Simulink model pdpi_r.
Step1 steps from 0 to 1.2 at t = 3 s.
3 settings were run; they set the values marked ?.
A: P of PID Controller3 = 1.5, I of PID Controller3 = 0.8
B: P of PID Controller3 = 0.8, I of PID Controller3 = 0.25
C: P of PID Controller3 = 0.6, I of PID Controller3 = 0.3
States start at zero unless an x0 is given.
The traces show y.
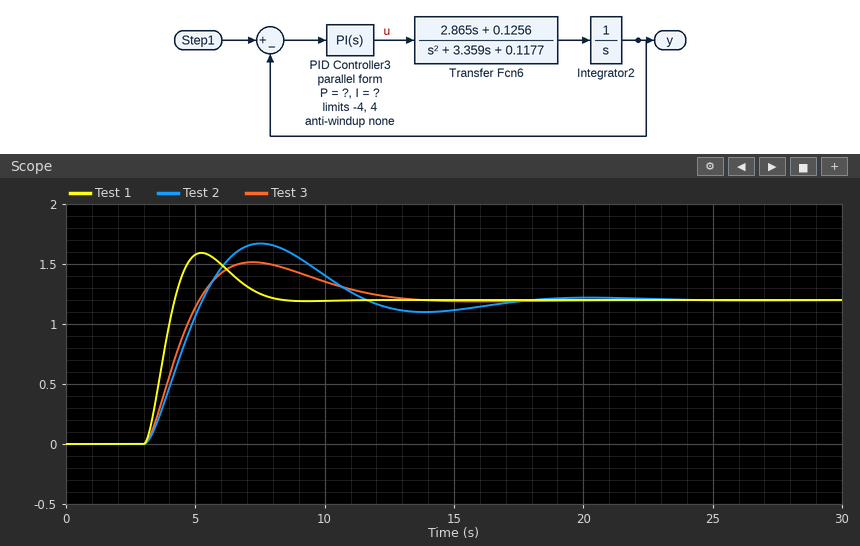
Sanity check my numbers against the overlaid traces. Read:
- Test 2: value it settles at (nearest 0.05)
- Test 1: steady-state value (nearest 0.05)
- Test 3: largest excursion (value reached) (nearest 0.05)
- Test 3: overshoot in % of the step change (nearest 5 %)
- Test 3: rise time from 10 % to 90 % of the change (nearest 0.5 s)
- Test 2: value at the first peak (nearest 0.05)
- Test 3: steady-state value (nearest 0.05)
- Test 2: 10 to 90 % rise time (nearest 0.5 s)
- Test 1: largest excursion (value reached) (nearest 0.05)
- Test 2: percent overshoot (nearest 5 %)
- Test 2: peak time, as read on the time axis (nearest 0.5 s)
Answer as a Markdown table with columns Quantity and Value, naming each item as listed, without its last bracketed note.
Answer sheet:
| Quantity | Value |
|---|---|
| Test 2: value it settles at | 1.20 |
| Test 1: steady-state value | 1.20 |
| Test 3: largest excursion (value reached) | 1.50 |
| Test 3: overshoot in % of the step change | 25 % |
| Test 3: rise time from 10 % to 90 % of the change | 1.5 s |
| Test 2: value at the first peak | 1.65 |
| Test 3: steady-state value | 1.20 |
| Test 2: 10 to 90 % rise time | 1.5 s |
| Test 1: largest excursion (value reached) | 1.60 |
| Test 2: percent overshoot | 40 % |
| Test 2: peak time, as read on the time axis | 7.5 s |
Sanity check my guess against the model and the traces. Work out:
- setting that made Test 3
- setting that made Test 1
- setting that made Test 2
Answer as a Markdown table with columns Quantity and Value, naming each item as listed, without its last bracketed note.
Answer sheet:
| Quantity | Value |
|---|---|
| setting that made Test 3 | B |
| setting that made Test 1 | A |
| setting that made Test 2 | C |
